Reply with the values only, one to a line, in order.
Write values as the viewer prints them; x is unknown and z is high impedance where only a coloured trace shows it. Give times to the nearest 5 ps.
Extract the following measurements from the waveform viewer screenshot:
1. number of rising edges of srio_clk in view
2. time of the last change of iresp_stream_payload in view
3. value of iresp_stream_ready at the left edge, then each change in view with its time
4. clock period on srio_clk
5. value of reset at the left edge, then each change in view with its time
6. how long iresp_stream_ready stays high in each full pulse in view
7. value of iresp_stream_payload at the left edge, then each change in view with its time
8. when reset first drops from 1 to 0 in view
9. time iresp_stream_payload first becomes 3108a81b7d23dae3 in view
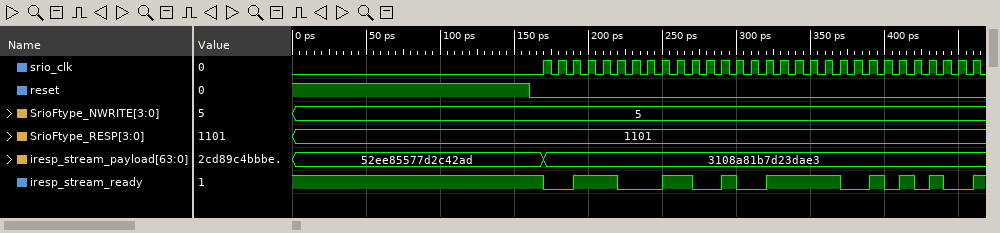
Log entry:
30
170 ps
1, 0 at 170 ps, 1 at 190 ps, 0 at 220 ps, 1 at 250 ps, 0 at 270 ps, 1 at 290 ps, 0 at 300 ps, 1 at 320 ps, 0 at 370 ps, 1 at 390 ps, 0 at 400 ps, 1 at 410 ps, 0 at 420 ps, 1 at 430 ps, 0 at 440 ps, 1 at 460 ps
10 ps
1, 0 at 160 ps
30 ps, 20 ps, 10 ps, 50 ps, 10 ps, 10 ps, 10 ps
52ee85577d2c42ad, 3108a81b7d23dae3 at 170 ps
160 ps
170 ps
